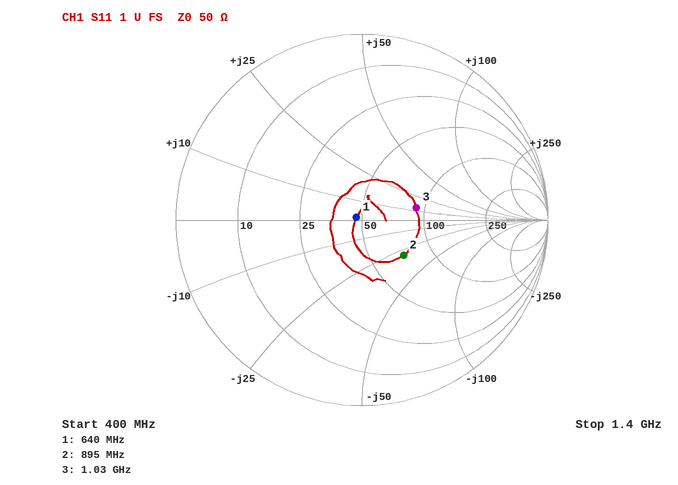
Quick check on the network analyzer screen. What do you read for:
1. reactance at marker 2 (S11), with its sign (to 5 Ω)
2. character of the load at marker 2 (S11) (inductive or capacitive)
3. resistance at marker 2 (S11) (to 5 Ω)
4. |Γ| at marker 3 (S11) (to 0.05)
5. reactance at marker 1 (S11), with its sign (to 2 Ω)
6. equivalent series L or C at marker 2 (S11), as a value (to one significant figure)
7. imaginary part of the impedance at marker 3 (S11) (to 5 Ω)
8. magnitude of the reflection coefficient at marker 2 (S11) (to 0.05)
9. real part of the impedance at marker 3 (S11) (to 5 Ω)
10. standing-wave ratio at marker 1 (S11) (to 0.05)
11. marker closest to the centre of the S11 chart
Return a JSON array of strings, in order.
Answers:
["-30 Ω", "capacitive", "70 Ω", "0.30", "+2 Ω", "6 pF", "+15 Ω", "0.30", "90 Ω", "1.05", "marker 1"]
